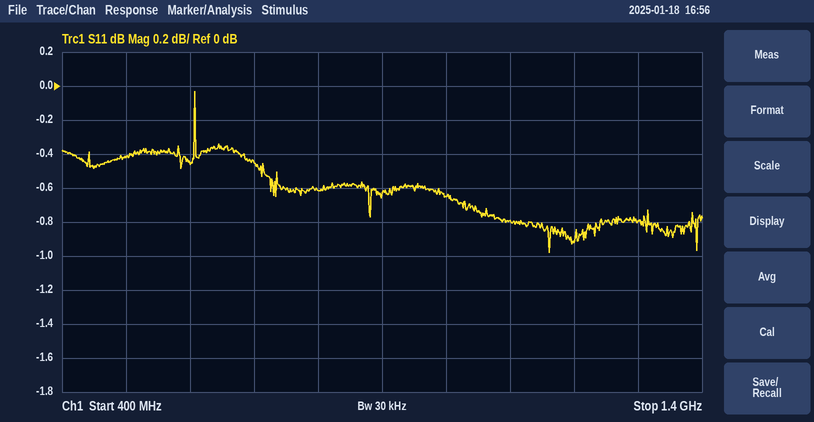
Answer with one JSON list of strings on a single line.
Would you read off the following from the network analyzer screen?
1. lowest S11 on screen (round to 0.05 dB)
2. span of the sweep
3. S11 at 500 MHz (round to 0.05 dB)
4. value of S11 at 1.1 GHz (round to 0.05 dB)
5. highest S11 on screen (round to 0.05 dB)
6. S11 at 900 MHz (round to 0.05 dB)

["-1.00 dB", "1 GHz", "-0.40 dB", "-0.80 dB", "-0.05 dB", "-0.65 dB"]
